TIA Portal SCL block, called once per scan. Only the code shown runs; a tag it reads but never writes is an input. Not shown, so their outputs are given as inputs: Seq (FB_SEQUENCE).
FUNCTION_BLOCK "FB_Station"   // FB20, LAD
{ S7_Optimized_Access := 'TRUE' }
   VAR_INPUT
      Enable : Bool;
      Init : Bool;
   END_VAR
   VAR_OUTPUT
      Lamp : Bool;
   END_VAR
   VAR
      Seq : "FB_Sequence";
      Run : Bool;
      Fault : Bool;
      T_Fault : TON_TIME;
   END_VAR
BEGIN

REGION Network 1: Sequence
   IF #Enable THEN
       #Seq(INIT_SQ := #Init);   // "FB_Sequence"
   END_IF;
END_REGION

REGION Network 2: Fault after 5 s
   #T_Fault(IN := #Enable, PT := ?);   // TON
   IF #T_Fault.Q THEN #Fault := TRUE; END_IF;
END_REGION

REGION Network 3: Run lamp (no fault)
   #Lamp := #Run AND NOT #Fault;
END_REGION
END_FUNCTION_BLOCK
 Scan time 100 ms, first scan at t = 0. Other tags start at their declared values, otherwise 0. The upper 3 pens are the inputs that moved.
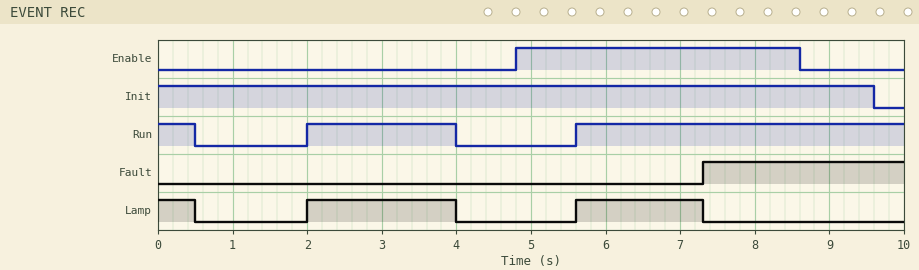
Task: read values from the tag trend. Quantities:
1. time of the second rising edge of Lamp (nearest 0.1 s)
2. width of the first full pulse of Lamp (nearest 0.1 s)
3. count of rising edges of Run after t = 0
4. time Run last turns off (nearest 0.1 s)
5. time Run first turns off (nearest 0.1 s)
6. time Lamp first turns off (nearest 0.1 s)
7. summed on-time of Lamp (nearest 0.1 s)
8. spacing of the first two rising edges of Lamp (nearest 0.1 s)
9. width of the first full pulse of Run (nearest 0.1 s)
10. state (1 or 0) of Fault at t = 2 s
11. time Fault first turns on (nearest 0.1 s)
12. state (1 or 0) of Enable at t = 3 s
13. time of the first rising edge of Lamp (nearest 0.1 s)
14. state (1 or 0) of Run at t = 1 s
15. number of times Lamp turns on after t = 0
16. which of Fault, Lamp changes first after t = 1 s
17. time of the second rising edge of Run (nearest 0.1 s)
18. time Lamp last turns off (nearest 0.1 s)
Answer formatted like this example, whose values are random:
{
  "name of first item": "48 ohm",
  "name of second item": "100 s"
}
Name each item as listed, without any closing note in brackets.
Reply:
{
  "time of the second rising edge of Lamp": "5.6 s",
  "width of the first full pulse of Lamp": "2.0 s",
  "count of rising edges of Run after t = 0": "2",
  "time Run last turns off": "4.0 s",
  "time Run first turns off": "0.5 s",
  "time Lamp first turns off": "0.5 s",
  "summed on-time of Lamp": "4.2 s",
  "spacing of the first two rising edges of Lamp": "3.6 s",
  "width of the first full pulse of Run": "2.0 s",
  "state (1 or 0) of Fault at t = 2 s": "0",
  "time Fault first turns on": "7.3 s",
  "state (1 or 0) of Enable at t = 3 s": "0",
  "time of the first rising edge of Lamp": "2.0 s",
  "state (1 or 0) of Run at t = 1 s": "0",
  "number of times Lamp turns on after t = 0": "2",
  "which of Fault, Lamp changes first after t = 1 s": "Lamp",
  "time of the second rising edge of Run": "5.6 s",
  "time Lamp last turns off": "7.3 s"
}
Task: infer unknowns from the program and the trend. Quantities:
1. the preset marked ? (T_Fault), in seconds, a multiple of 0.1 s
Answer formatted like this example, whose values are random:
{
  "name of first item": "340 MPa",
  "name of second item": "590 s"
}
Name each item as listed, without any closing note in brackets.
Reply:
{
  "the preset marked ? (T_Fault), in seconds, a multiple of 0.1 s": "2.5 s"
}
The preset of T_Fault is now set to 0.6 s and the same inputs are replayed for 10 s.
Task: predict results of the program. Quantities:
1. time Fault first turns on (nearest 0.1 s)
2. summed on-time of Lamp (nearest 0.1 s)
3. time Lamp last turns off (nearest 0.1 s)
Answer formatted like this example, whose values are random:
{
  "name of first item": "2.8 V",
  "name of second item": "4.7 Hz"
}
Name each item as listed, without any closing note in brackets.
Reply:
{
  "time Fault first turns on": "5.4 s",
  "summed on-time of Lamp": "2.5 s",
  "time Lamp last turns off": "4.0 s"
}
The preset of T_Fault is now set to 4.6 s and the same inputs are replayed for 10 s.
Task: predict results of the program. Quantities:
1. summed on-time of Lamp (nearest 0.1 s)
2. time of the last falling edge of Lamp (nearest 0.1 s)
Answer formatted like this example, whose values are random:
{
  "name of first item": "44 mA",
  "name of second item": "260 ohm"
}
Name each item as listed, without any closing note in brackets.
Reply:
{
  "summed on-time of Lamp": "6.9 s",
  "time of the last falling edge of Lamp": "4.0 s"
}
